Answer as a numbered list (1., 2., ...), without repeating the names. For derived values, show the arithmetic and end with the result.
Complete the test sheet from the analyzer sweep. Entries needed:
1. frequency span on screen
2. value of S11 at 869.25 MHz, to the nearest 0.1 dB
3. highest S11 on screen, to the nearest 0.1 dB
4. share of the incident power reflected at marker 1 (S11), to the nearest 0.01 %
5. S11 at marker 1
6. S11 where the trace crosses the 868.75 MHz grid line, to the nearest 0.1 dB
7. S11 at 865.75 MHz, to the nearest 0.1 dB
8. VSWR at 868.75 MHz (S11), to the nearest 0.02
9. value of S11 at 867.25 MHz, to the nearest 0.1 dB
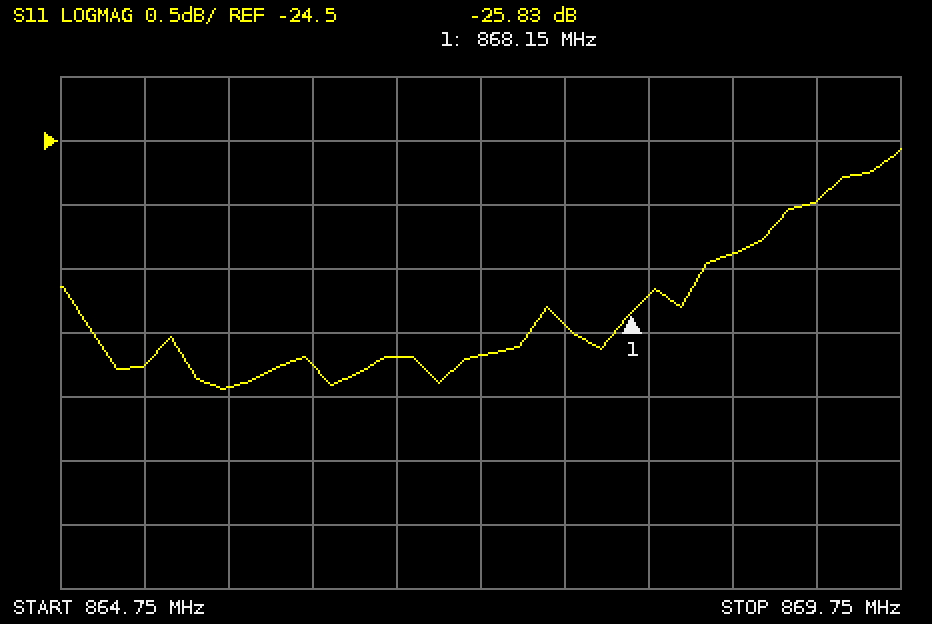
1. 5 MHz
2. -25.0 dB
3. -24.6 dB
4. 10^(-25.83/10) ≈ 0.26 %
5. -25.83 dB
6. -25.4 dB
7. -26.4 dB
8. |Γ| = 10^(-25.4/20) = 0.0537; VSWR = (1 + 0.0537)/(1 − 0.0537) ≈ 1.11, so 1.12 to the nearest 0.02
9. -26.2 dB
